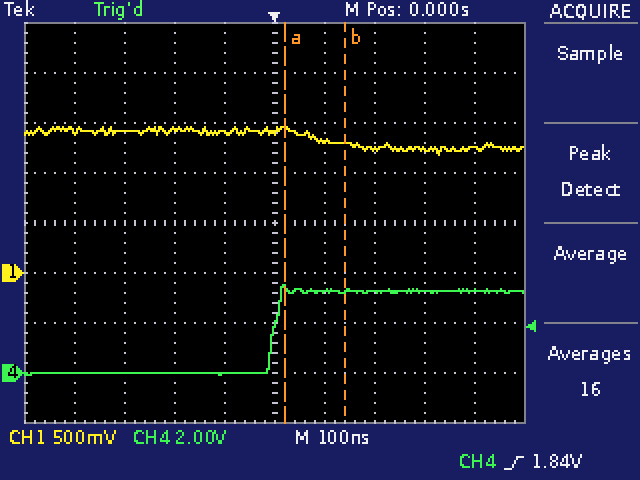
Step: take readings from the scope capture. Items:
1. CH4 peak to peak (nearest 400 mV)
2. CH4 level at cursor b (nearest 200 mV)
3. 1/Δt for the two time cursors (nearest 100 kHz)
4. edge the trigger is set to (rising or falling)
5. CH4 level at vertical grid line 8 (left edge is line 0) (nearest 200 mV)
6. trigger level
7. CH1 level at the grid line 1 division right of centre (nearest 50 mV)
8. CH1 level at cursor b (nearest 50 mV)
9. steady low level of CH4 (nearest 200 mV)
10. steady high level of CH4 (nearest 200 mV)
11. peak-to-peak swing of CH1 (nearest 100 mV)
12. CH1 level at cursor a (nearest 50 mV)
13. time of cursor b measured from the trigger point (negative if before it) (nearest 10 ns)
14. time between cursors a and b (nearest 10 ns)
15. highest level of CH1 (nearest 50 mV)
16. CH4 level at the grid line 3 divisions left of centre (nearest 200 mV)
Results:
3.6 V
3.2 V
8.3 MHz
rising
3.2 V
1.84 V
1.30 V
1.30 V
0.0 V
3.2 V
300 mV
1.45 V
+140 ns
120 ns
1.45 V
0.0 V
